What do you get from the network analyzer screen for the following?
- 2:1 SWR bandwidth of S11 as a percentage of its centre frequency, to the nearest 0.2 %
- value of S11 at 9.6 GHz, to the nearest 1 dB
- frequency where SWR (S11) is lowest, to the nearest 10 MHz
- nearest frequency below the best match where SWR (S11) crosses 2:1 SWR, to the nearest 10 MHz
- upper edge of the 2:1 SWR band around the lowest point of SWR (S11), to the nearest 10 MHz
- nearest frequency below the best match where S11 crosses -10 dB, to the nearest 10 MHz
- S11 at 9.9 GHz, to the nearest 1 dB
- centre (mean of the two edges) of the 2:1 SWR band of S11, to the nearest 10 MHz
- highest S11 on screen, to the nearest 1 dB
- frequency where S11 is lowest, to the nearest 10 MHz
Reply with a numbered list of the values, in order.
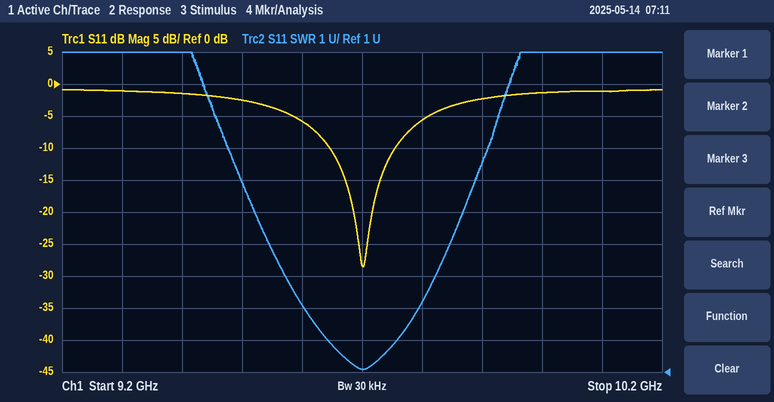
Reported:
1. 1.2 %
2. -6 dB
3. 9.70 GHz
4. 9.64 GHz
5. 9.76 GHz
6. 9.65 GHz
7. -2 dB
8. 9.70 GHz
9. -1 dB
10. 9.70 GHz
